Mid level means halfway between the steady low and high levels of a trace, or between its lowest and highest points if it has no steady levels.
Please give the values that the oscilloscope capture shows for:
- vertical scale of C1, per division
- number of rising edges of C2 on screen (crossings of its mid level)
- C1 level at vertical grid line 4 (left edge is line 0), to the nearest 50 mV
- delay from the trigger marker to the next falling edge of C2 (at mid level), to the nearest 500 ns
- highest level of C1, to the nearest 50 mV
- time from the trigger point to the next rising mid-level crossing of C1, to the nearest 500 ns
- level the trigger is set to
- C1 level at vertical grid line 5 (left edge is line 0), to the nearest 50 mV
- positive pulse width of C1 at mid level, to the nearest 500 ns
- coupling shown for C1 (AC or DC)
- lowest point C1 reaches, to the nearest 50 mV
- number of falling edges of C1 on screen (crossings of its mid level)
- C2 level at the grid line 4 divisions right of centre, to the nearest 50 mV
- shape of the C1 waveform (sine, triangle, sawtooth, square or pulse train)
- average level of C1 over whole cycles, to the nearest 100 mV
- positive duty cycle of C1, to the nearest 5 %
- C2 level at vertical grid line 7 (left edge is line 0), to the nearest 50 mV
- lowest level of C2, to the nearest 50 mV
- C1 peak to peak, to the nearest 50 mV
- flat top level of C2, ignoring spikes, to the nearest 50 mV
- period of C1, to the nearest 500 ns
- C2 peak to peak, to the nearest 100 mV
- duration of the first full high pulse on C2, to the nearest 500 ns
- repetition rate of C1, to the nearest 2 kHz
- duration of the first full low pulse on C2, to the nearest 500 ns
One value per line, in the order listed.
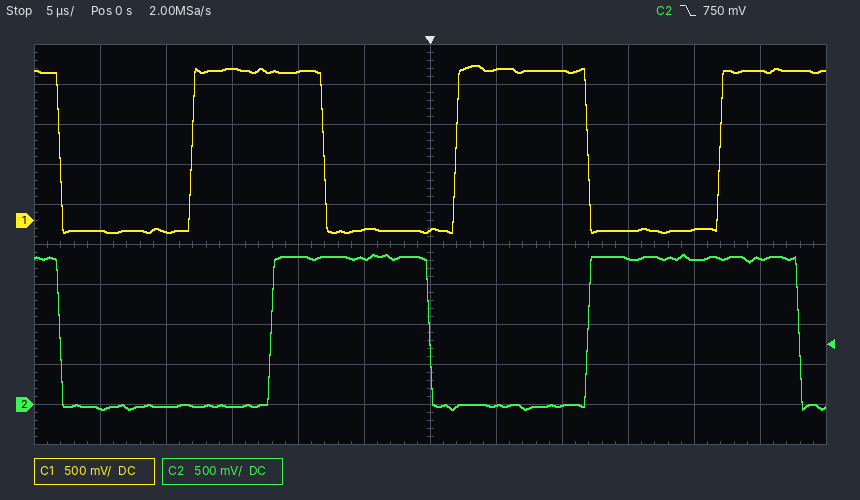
500 mV
2
1.85 V
28.0 µs
1.95 V
2.0 µs
750 mV
-100 mV
10.0 µs
DC
-150 mV
3
1.80 V
square
900 mV
50 %
0 mV
-50 mV
2.10 V
1.85 V
20.0 µs
1.90 V
12.0 µs
50 kHz
16.0 µs
